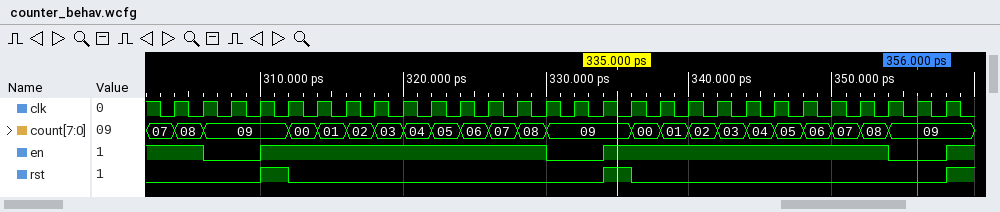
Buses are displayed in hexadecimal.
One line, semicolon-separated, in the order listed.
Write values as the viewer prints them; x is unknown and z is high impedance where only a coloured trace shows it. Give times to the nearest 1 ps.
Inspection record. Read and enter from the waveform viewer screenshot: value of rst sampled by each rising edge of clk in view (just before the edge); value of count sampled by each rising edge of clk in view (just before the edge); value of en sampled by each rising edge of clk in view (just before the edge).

0 0 0 0 1 0 0 0 0 0 0 0 0 0 0 0 1 0 0 0 0 0 0 0 0 0 0 0; 07, 08, 09, 09, 09, 00, 01, 02, 03, 04, 05, 06, 07, 08, 09, 09, 09, 00, 01, 02, 03, 04, 05, 06, 07, 08, 09, 09; 1 1 0 0 1 1 1 1 1 1 1 1 1 1 0 0 1 1 1 1 1 1 1 1 1 1 0 0
